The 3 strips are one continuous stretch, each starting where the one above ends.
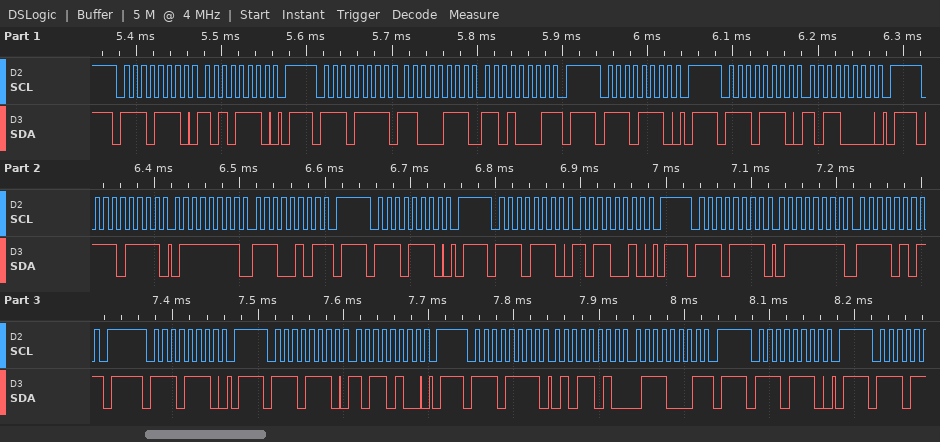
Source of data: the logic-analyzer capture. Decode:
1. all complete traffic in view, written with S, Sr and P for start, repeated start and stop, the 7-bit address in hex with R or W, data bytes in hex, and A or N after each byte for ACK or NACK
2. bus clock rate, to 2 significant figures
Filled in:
S 77W A AE A P S 77R A C7 A D1 N P S 77W A P S 77W A B0 A P S 77R A 7F A E5 N P S 77W A P S 77W A B2 A P S 77R A 7F A F5 N P S 77W A P S 77W A B4 A P S 77R A 5A A 71 N P S 77W A P
100 kHz
